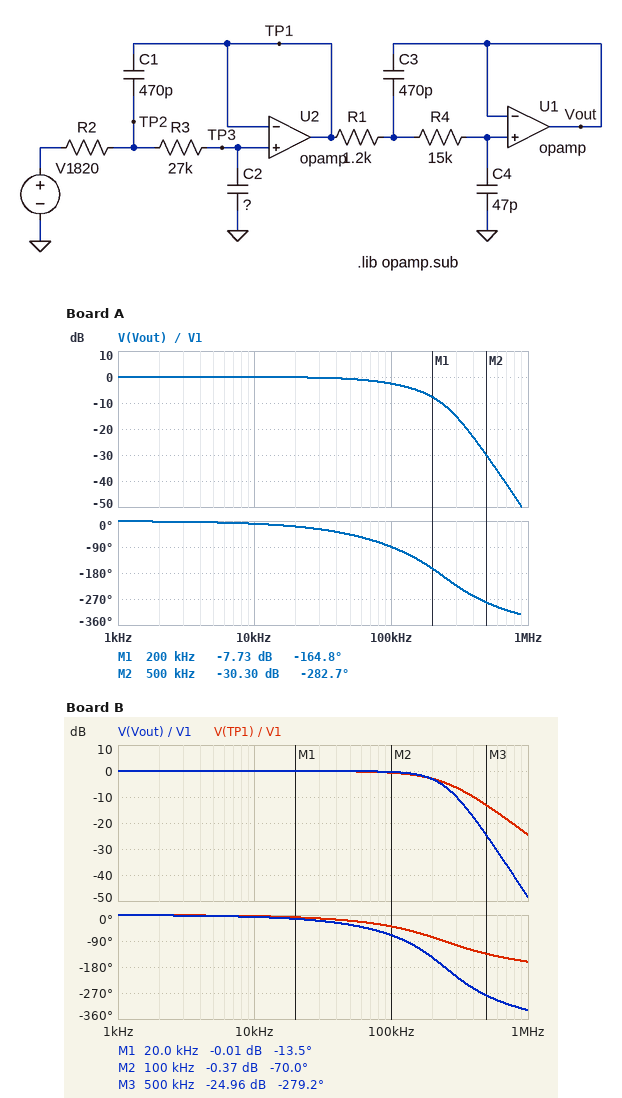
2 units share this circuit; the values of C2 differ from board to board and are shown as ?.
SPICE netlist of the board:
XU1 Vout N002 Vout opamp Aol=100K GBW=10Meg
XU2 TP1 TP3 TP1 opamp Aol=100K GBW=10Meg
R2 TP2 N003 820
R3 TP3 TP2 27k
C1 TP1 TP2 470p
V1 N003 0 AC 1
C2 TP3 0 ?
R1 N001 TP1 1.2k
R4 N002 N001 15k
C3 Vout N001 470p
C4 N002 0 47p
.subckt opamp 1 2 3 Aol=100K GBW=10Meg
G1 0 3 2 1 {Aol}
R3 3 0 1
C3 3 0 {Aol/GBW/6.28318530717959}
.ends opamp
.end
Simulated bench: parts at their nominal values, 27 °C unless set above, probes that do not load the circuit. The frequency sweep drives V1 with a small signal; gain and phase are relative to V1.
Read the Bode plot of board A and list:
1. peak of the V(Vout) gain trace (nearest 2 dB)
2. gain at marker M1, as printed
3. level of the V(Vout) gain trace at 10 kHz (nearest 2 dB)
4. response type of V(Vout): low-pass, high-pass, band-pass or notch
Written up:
0 dB
-7.73 dB
0 dB
low-pass
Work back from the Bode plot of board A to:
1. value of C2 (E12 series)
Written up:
68 pF
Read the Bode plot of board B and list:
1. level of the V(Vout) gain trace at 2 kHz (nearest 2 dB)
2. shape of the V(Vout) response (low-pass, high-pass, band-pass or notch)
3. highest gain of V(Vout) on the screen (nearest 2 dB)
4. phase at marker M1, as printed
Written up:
0 dB
low-pass
0 dB
-13.5 deg
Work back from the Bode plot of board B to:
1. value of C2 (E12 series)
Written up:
39 pF
